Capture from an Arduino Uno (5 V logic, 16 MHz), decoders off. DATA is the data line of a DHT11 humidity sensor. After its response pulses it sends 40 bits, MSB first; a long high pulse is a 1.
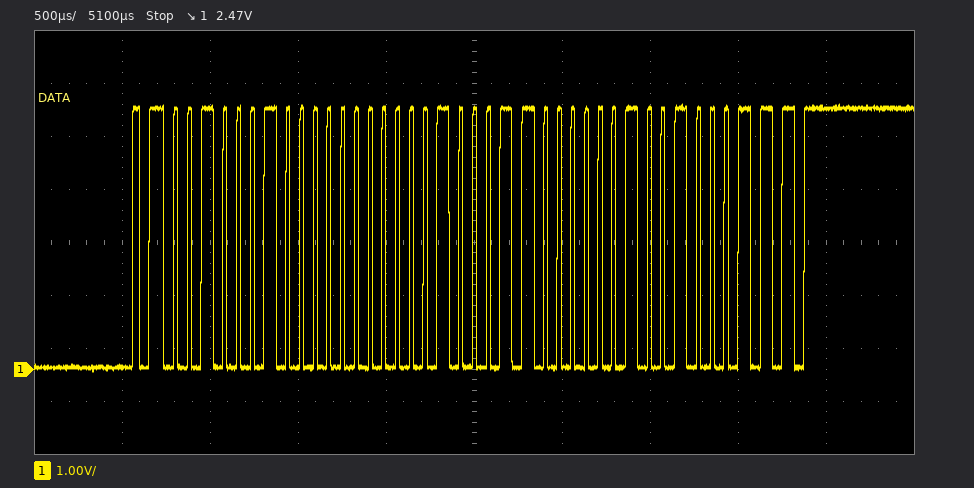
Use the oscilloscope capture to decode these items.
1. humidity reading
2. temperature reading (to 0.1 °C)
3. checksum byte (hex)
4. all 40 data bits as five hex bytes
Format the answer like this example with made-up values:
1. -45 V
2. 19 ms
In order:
1. 34 %
2. 35.2 °C
3. 0x47
4. 22 00 23 02 47
